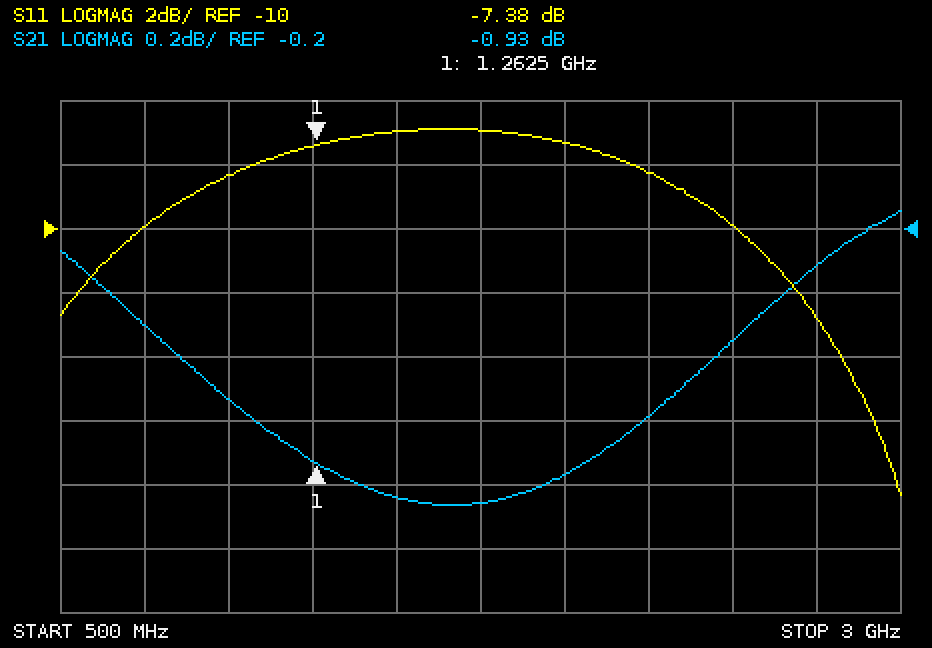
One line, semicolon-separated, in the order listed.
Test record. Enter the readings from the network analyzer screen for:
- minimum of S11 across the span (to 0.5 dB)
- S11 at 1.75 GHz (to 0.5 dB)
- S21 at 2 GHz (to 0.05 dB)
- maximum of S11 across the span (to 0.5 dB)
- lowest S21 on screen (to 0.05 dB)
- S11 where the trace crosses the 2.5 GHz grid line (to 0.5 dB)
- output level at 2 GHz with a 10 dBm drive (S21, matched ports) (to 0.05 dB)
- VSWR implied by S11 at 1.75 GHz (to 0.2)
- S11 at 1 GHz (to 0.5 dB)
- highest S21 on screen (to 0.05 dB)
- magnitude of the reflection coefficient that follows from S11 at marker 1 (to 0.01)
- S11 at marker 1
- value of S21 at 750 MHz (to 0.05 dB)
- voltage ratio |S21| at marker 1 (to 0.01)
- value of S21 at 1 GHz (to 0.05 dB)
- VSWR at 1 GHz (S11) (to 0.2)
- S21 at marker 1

-18.5 dB; -7.0 dB; -0.95 dB; -7.0 dB; -1.05 dB; -10.0 dB; 9.05 dBm; 2.6; -8.5 dB; -0.15 dB; 0.43; -7.38 dB; -0.50 dB; 0.90; -0.75 dB; 2.2; -0.93 dB
